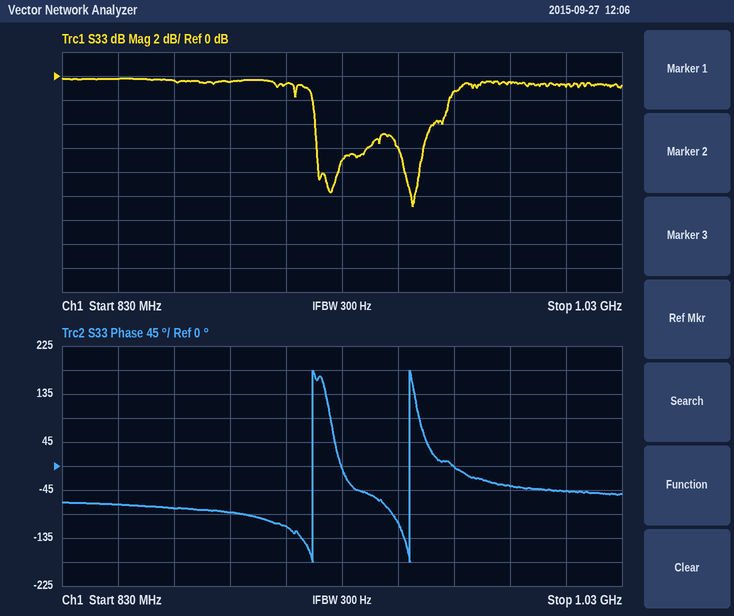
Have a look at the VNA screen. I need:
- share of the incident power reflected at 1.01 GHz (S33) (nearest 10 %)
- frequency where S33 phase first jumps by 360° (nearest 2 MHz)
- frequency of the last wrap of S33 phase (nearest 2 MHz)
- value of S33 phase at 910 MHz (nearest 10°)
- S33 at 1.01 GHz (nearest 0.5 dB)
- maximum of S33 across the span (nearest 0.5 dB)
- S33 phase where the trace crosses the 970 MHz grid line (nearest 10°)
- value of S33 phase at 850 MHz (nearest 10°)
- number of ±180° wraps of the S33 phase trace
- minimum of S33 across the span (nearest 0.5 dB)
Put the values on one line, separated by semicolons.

80 %; 920 MHz; 954 MHz; -110°; -1.0 dB; 0.0 dB; 0°; -70°; 2; -11.0 dB
